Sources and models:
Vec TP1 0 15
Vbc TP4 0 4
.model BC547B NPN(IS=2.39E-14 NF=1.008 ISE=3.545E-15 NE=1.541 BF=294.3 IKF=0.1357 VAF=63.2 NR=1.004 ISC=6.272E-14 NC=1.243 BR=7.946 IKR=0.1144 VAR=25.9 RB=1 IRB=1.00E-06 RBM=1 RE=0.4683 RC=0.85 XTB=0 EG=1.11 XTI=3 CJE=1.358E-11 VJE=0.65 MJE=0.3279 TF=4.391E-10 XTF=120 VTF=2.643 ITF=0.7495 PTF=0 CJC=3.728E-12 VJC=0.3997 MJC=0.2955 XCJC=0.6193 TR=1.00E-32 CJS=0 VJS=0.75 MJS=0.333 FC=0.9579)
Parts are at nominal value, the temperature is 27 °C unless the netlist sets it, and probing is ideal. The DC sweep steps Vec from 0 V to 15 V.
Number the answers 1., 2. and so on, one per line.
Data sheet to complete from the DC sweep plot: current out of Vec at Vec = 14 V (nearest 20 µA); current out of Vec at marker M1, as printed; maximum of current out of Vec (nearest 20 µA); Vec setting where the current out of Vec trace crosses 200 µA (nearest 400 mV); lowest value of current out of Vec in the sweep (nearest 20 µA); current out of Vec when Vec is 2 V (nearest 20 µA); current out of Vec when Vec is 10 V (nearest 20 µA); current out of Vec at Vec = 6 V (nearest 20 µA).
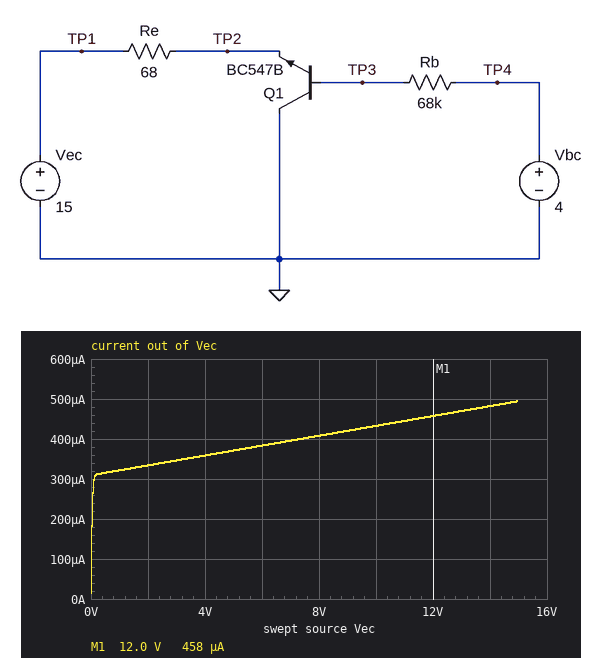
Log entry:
1. 480 µA
2. 458 µA
3. 500 µA
4. 0 V
5. 20 µA
6. 340 µA
7. 440 µA
8. 380 µA
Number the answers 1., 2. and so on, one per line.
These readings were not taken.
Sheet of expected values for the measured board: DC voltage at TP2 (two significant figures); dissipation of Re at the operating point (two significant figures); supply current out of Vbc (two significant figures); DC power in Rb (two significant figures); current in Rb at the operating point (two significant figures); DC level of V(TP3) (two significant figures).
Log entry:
1. 15 V
2. 17 µW
3. 50 µA
4. 170 µW
5. 50 µA
6. 610 mV
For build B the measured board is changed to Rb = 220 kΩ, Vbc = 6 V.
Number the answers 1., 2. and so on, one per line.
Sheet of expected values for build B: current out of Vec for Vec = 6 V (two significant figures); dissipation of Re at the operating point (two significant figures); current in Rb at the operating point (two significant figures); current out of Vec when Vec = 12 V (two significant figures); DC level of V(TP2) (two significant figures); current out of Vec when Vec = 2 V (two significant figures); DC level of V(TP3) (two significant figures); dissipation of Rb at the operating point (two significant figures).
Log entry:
1. 180 µA
2. 3.8 µW
3. 25 µA
4. 220 µA
5. 15 V
6. 160 µA
7. 590 mV
8. 130 µW
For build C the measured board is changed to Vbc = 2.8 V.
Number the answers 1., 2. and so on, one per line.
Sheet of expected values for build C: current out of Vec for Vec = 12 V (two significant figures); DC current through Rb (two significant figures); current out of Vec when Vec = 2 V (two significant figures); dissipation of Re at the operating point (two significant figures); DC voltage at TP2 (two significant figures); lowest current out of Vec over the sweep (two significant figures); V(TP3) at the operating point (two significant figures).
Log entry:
1. 290 µA
2. 32 µA
3. 210 µA
4. 6.8 µW
5. 15 V
6. 11 µA
7. 590 mV
